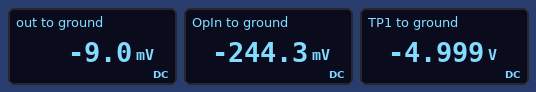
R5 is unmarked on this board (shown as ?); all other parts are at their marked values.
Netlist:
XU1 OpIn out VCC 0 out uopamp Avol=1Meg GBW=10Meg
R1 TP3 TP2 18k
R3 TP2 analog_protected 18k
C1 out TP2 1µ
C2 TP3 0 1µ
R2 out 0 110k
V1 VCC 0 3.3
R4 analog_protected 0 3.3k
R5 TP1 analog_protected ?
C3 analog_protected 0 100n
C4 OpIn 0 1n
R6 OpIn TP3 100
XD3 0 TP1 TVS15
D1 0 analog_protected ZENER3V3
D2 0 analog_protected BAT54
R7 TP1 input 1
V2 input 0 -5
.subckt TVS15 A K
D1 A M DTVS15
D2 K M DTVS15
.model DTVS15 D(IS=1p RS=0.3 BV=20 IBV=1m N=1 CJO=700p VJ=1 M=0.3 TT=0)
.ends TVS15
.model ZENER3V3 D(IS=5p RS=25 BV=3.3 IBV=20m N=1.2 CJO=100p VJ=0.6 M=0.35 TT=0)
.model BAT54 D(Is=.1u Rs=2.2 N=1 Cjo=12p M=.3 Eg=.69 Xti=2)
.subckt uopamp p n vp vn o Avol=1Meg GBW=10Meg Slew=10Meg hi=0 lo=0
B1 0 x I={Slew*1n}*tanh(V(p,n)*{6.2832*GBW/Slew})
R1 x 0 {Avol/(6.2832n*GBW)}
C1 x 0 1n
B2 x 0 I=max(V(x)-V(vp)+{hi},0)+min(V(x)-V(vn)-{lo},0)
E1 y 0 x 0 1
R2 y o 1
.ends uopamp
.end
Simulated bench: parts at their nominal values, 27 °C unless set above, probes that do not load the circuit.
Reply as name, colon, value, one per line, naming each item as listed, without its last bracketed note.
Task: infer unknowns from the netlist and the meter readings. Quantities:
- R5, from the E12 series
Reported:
R5, from the E12 series: 3.9 kΩ
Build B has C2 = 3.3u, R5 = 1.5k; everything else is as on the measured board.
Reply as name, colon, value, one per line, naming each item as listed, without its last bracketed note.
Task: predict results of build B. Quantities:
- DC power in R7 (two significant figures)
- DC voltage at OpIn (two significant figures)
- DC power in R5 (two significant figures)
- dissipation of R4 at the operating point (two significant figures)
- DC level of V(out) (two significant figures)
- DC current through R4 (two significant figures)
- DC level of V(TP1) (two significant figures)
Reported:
DC power in R7: 9.9 µW
DC voltage at OpIn: -270 mV
DC power in R5: 15 mW
dissipation of R4 at the operating point: 23 µW
DC level of V(out): -9.3 mV
DC current through R4: 83 µA
DC level of V(TP1): -5.0 V
